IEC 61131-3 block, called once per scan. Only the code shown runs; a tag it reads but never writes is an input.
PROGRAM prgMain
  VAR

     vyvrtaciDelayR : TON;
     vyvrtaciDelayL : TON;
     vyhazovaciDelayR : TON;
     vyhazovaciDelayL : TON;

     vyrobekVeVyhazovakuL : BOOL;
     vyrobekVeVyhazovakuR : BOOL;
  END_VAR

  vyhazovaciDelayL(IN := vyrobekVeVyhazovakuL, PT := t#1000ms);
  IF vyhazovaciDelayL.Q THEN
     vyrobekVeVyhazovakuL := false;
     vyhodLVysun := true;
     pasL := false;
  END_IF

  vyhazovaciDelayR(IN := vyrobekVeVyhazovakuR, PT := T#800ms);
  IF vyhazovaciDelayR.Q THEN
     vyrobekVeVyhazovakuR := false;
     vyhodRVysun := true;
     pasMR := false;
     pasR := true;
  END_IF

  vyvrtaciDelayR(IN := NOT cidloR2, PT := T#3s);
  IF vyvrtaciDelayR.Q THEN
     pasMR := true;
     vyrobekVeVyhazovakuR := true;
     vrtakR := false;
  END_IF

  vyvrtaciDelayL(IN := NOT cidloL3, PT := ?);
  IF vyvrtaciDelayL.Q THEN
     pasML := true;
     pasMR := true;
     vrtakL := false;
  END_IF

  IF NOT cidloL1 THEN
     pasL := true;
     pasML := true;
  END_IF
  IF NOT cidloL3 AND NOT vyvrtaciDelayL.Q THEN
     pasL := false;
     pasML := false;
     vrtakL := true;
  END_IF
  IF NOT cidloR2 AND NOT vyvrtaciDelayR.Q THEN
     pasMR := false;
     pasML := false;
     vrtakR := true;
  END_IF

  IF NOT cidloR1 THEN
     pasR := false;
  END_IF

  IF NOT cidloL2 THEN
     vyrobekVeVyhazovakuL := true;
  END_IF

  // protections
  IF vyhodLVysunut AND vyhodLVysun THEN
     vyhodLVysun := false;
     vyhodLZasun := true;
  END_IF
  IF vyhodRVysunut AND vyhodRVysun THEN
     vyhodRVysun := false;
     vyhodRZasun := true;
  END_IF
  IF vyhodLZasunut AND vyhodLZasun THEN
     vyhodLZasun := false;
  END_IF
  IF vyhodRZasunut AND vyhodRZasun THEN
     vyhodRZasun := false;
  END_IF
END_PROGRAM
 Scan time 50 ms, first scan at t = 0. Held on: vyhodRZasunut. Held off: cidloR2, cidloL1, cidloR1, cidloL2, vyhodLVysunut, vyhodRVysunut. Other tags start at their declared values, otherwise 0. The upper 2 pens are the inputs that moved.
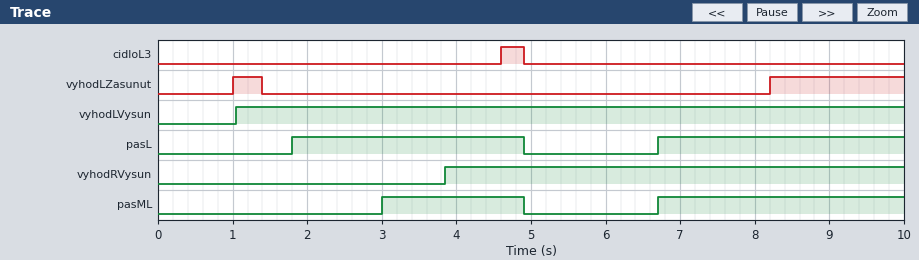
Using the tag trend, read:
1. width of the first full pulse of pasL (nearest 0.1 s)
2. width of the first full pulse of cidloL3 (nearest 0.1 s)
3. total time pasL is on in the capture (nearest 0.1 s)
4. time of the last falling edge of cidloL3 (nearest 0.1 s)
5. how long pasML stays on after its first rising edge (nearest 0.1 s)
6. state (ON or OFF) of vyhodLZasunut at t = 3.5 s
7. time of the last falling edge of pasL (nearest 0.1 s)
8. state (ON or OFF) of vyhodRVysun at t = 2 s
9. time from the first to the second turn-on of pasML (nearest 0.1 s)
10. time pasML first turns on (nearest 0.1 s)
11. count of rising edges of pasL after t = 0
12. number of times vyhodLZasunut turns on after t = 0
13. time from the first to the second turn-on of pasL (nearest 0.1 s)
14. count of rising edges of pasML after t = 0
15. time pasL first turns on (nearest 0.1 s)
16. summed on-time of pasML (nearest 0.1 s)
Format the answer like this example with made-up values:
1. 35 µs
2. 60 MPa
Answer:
1. 3.1 s
2. 0.3 s
3. 6.4 s
4. 4.9 s
5. 1.9 s
6. OFF
7. 4.9 s
8. OFF
9. 3.7 s
10. 3.0 s
11. 2
12. 2
13. 4.9 s
14. 2
15. 1.8 s
16. 5.2 s
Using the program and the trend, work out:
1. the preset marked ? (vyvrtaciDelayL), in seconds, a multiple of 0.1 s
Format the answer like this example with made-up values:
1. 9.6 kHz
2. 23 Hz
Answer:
1. 1.8 s
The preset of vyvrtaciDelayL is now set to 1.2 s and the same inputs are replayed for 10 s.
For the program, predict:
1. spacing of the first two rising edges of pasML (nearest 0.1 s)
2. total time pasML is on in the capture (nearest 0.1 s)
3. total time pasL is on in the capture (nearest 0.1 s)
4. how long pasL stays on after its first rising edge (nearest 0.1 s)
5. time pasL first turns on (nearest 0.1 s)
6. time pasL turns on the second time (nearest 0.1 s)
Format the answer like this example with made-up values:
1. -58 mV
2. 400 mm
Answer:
1. 3.1 s
2. 5.8 s
3. 7.6 s
4. 3.7 s
5. 1.2 s
6. 6.1 s
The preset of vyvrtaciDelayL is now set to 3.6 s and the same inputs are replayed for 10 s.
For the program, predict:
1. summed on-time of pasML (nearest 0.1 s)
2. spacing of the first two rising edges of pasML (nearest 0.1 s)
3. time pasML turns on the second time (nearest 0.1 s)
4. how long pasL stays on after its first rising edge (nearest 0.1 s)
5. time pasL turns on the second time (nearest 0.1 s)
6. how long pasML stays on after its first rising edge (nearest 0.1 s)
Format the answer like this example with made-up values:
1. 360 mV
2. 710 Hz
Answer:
1. 2.8 s
2. 4.9 s
3. 8.5 s
4. 1.3 s
5. 8.5 s
6. 1.3 s
